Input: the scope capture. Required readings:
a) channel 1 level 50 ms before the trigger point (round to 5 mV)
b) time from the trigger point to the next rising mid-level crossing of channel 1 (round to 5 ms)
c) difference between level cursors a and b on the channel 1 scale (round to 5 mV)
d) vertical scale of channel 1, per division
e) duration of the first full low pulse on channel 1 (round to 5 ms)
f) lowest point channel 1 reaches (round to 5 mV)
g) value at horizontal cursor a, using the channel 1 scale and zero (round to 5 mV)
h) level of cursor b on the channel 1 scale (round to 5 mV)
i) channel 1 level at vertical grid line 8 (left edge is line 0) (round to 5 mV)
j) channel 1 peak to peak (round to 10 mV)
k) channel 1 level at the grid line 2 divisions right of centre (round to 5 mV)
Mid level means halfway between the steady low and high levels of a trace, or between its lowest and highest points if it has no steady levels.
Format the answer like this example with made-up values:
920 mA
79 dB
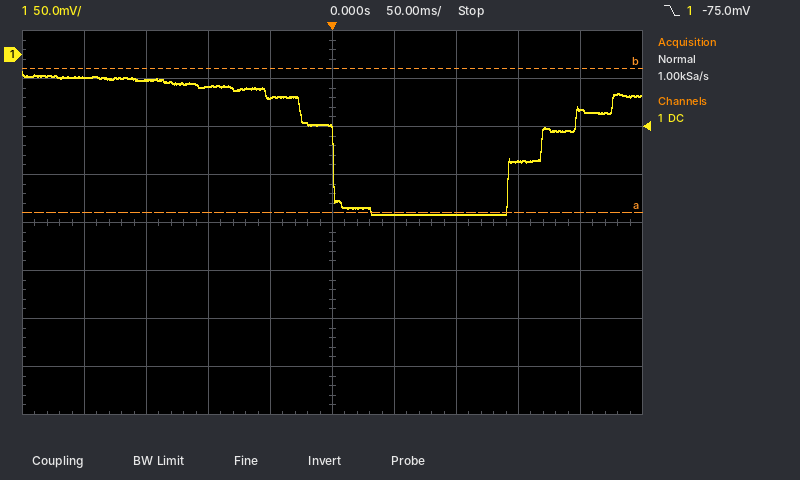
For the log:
-45 mV
170 ms
150 mV
50 mV
170 ms
-165 mV
-165 mV
-15 mV
-110 mV
150 mV
-165 mV
